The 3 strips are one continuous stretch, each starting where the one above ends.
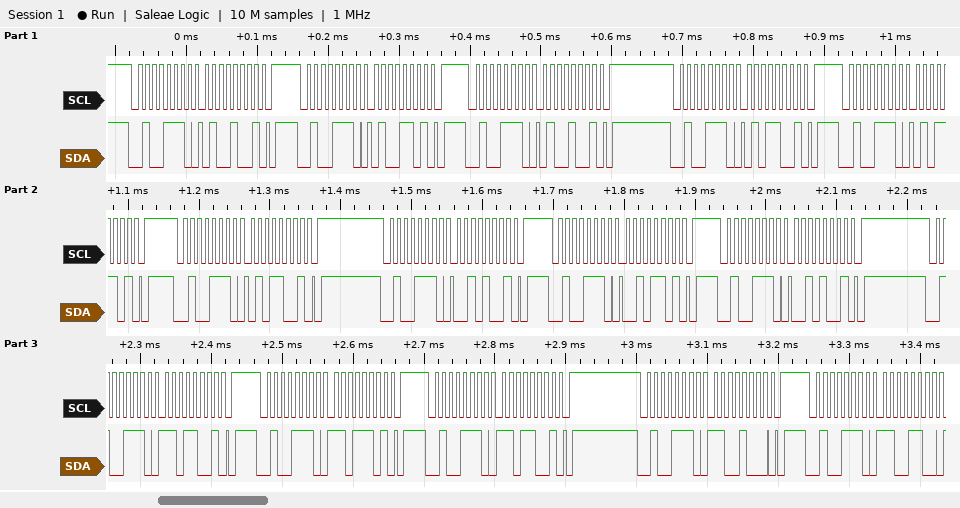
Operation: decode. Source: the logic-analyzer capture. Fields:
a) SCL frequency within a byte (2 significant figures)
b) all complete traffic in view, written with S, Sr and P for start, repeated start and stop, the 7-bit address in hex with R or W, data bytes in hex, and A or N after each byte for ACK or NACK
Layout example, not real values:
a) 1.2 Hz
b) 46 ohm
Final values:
a) 100 kHz
b) S 27W A 49 A P S 27W A 4D A P S 27W A 49 A P S 27W A 59 A P S 27W A 5D A P S 27W A 59 A P S 27W A 29 A P S 27W A 2D A P S 27W A 29 A P S 27W A D9 A P S 27W A DD A P S 27W A D9 A P S 27W A C8 A P S 27W A CC A
